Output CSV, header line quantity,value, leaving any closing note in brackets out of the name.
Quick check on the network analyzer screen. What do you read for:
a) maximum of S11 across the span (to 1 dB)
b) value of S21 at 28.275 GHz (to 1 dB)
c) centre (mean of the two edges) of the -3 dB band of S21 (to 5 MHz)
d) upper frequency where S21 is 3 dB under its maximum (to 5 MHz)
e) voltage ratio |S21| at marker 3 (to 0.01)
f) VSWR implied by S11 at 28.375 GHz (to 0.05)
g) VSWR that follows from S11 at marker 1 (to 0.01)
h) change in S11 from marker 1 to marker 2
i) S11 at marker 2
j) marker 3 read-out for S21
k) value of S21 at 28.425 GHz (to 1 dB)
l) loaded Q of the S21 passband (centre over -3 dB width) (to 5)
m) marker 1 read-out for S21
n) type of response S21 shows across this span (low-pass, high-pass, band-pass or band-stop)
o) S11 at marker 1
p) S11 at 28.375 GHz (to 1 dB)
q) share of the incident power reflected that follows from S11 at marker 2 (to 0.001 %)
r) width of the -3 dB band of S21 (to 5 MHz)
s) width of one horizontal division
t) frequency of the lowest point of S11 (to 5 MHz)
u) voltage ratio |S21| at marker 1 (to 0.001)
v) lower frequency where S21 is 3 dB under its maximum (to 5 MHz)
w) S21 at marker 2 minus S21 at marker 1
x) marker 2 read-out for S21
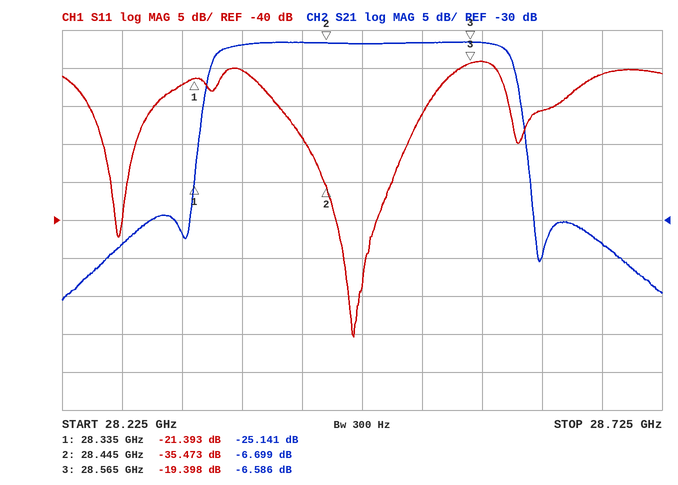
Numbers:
quantity,value
maximum of S11 across the span,-19 dB
value of S21 at 28.275 GHz,-33 dB
centre (mean of the two edges) of the -3 dB band of S21,28.475 GHz
upper frequency where S21 is 3 dB under its maximum,28.600 GHz
voltage ratio |S21| at marker 3,0.47
VSWR implied by S11 at 28.375 GHz,1.20
VSWR that follows from S11 at marker 1,1.19
change in S11 from marker 1 to marker 2,-14.080 dB
S11 at marker 2,-35.473 dB
marker 3 read-out for S21,-6.586 dB
value of S21 at 28.425 GHz,-7 dB
loaded Q of the S21 passband (centre over -3 dB width),115
marker 1 read-out for S21,-25.141 dB
type of response S21 shows across this span,band-pass
S11 at marker 1,-21.393 dB
S11 at 28.375 GHz,-20 dB
share of the incident power reflected that follows from S11 at marker 2,0.028 %
width of the -3 dB band of S21,250 MHz
width of one horizontal division,50 MHz
frequency of the lowest point of S11,28.470 GHz
voltage ratio |S21| at marker 1,0.055
lower frequency where S21 is 3 dB under its maximum,28.350 GHz
S21 at marker 2 minus S21 at marker 1,18.442 dB
marker 2 read-out for S21,-6.699 dB
